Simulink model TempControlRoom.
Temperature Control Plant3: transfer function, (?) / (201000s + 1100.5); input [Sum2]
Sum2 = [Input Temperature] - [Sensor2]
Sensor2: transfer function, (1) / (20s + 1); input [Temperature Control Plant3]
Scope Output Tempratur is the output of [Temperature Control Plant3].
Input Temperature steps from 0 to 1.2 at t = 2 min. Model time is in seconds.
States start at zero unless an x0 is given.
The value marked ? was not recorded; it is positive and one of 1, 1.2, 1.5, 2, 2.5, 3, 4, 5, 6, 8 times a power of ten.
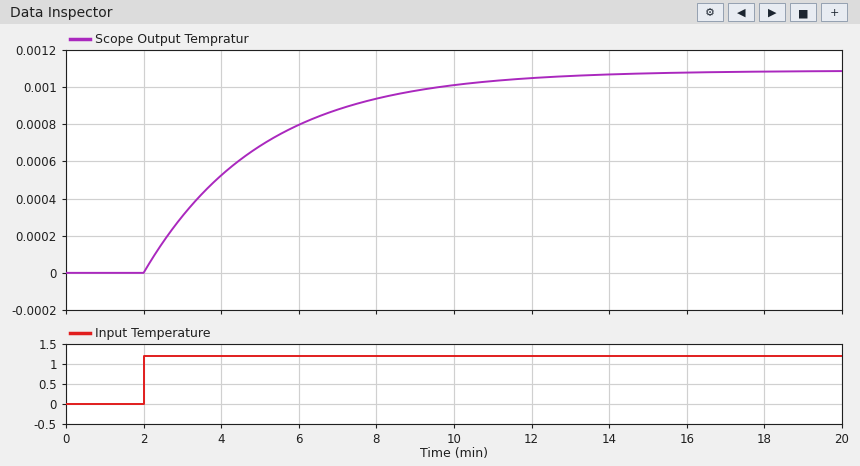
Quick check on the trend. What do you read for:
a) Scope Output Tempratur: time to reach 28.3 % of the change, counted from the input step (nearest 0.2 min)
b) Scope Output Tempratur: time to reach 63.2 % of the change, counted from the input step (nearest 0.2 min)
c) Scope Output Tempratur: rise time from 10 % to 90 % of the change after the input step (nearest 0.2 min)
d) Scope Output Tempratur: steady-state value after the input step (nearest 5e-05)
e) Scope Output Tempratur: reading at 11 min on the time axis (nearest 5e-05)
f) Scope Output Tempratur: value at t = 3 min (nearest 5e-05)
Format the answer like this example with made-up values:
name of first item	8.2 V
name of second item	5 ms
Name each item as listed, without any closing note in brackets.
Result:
Scope Output Tempratur: time to reach 28.3 % of the change, counted from the input step	1.0 min
Scope Output Tempratur: time to reach 63.2 % of the change, counted from the input step	3.0 min
Scope Output Tempratur: rise time from 10 % to 90 % of the change after the input step	6.6 min
Scope Output Tempratur: steady-state value after the input step	0.00110
Scope Output Tempratur: reading at 11 min on the time axis	0.00105
Scope Output Tempratur: value at t = 3 min	0.00030
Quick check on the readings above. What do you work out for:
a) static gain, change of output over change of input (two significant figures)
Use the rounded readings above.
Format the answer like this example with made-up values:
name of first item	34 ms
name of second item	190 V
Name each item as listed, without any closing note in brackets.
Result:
static gain, change of output over change of input	0.00092
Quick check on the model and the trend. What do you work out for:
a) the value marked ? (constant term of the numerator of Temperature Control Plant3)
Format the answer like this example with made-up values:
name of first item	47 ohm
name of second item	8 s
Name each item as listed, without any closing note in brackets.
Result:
the value marked ?	1
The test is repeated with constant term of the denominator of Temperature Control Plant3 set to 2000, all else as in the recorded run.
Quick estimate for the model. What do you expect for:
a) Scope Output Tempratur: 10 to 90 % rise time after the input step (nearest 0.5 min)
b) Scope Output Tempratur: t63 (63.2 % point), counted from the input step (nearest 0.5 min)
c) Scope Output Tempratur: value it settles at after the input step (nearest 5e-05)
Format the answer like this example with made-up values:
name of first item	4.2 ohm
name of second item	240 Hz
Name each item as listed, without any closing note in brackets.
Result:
Scope Output Tempratur: 10 to 90 % rise time after the input step	3.5 min
Scope Output Tempratur: t63 (63.2 % point), counted from the input step	1.5 min
Scope Output Tempratur: value it settles at after the input step	0.00060
